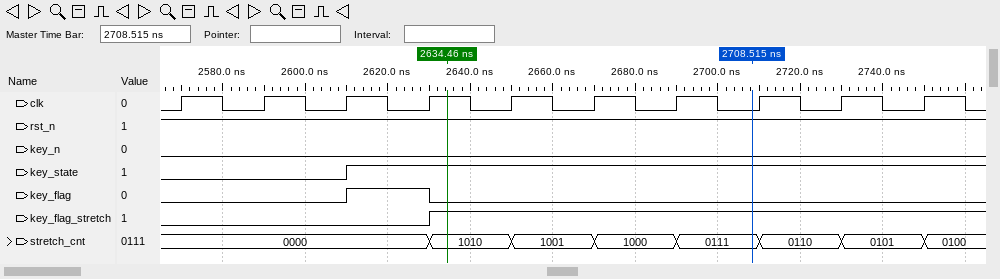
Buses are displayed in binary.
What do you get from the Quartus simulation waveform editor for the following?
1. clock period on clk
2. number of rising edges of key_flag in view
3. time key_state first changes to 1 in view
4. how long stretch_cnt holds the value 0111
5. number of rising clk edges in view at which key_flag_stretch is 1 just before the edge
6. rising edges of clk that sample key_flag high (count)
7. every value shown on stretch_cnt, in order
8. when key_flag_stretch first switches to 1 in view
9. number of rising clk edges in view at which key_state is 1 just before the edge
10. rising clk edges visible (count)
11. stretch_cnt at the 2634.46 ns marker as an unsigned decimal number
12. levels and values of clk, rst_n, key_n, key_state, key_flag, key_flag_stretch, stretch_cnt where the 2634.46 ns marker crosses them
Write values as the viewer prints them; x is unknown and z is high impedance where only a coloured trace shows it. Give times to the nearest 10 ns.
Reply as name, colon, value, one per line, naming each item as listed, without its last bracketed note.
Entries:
clock period on clk: 20 ns
number of rising edges of key_flag in view: 1
time key_state first changes to 1 in view: 2610 ns
how long stretch_cnt holds the value 0111: 20 ns
number of rising clk edges in view at which key_flag_stretch is 1 just before the edge: 6
rising edges of clk that sample key_flag high: 1
every value shown on stretch_cnt, in order: 0000, 1010, 1001, 1000, 0111, 0110, 0101, 0100
when key_flag_stretch first switches to 1 in view: 2630 ns
number of rising clk edges in view at which key_state is 1 just before the edge: 7
rising clk edges visible: 10
stretch_cnt at the 2634.46 ns marker as an unsigned decimal number: 10
levels and values of clk, rst_n, key_n, key_state, key_flag, key_flag_stretch, stretch_cnt where the 2634.46 ns marker crosses them: clk=1, rst_n=1, key_n=0, key_state=1, key_flag=0, key_flag_stretch=1, stretch_cnt=1010
